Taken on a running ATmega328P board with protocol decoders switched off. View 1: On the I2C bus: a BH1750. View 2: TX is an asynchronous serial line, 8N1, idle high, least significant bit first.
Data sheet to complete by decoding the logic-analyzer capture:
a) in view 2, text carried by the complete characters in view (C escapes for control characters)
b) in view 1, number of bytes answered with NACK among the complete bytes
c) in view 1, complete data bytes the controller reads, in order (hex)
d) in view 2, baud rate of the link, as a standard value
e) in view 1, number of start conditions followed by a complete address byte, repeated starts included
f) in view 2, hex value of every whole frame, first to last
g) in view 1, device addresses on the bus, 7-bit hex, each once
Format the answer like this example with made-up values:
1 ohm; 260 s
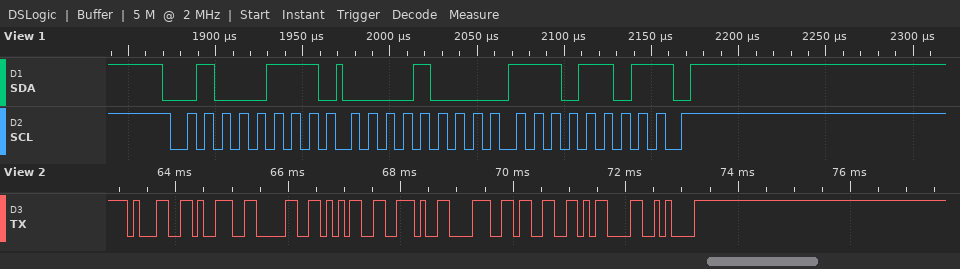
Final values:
"1905.83\r\n"; 1; 08 ED; 9600 baud; 1; 31 39 30 35 2E 38 33 0D 0A; 0x23
